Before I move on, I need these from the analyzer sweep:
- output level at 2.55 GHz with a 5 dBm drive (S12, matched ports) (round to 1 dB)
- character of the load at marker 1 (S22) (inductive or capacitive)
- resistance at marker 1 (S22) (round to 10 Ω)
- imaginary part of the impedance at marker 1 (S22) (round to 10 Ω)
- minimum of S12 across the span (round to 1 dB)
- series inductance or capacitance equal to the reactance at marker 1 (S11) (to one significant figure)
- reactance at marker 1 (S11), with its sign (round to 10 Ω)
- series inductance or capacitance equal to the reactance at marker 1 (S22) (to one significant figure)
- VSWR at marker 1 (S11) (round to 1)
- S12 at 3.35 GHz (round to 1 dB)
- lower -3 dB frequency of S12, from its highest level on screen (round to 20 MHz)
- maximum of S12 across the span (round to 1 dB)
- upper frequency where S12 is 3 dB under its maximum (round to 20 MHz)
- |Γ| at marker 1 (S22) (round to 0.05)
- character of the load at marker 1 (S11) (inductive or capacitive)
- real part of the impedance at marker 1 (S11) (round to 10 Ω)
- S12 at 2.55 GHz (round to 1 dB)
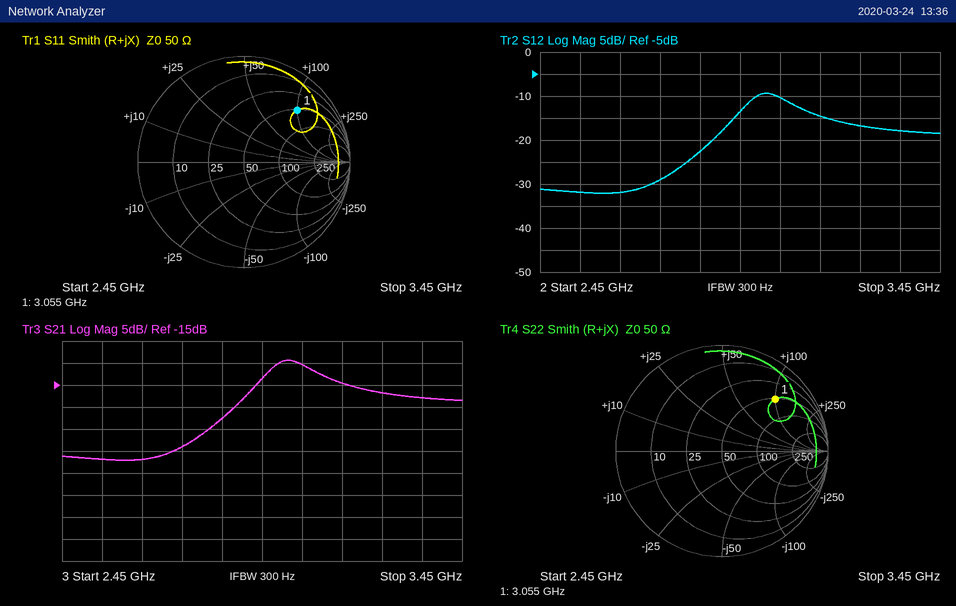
-27 dBm
inductive
50 Ω
+100 Ω
-32 dB
5 nH
+100 Ω
5 nH
6
-18 dB
2.96 GHz
-9 dB
3.10 GHz
0.70
inductive
50 Ω
-32 dB
